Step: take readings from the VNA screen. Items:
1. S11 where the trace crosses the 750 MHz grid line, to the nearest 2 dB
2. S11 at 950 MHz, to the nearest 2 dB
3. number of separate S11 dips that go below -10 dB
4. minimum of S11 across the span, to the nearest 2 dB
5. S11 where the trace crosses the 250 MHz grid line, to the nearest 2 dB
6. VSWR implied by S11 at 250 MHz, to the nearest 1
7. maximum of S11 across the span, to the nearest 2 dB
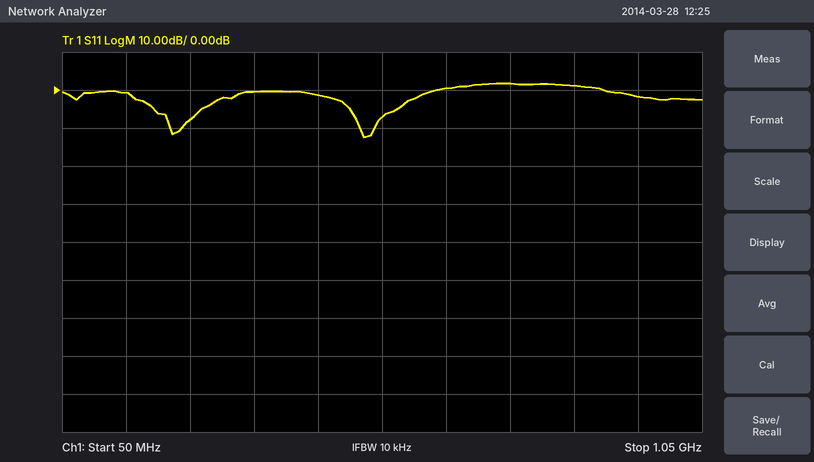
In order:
2 dB
-2 dB
2
-12 dB
-8 dB
2
2 dB
